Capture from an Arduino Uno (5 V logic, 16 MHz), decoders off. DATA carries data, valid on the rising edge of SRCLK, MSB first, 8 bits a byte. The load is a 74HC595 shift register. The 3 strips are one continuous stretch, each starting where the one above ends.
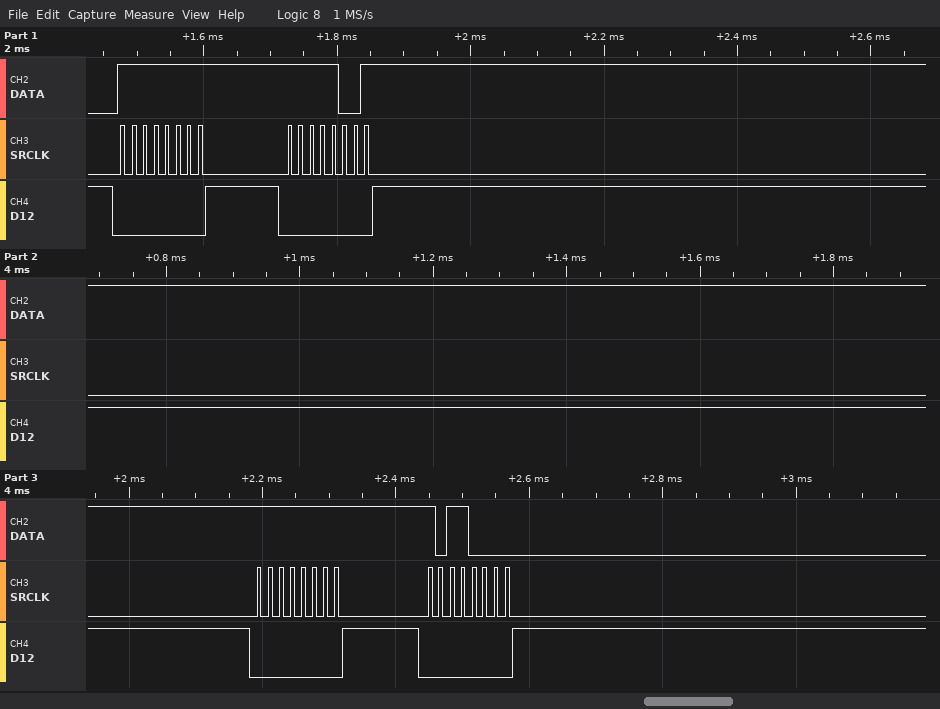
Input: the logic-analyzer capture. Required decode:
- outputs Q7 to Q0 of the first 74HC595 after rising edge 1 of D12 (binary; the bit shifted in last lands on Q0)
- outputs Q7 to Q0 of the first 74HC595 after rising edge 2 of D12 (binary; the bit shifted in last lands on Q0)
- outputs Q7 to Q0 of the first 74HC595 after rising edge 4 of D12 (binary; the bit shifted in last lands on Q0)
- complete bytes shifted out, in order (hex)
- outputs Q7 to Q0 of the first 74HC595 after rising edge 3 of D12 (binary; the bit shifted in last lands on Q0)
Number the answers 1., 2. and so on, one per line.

1. 11111111
2. 11111001
3. 10110000
4. 0xFF 0xF9 0xFF 0xB0
5. 11111111
